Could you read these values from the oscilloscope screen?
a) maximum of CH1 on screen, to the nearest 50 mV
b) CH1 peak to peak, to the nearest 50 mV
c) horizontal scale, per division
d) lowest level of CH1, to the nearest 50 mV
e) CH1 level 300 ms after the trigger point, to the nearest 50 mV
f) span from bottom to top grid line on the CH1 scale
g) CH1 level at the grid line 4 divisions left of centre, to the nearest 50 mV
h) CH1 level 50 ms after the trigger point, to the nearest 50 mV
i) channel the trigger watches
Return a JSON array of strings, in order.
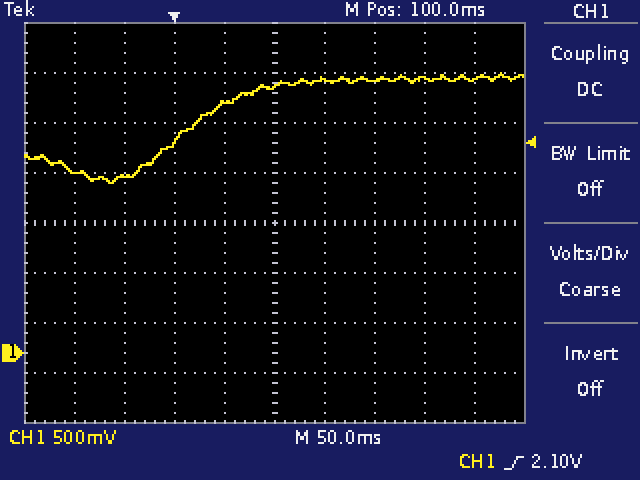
["2.80 V", "1.10 V", "50 ms", "1.70 V", "2.75 V", "4 V", "1.80 V", "2.50 V", "CH1"]
